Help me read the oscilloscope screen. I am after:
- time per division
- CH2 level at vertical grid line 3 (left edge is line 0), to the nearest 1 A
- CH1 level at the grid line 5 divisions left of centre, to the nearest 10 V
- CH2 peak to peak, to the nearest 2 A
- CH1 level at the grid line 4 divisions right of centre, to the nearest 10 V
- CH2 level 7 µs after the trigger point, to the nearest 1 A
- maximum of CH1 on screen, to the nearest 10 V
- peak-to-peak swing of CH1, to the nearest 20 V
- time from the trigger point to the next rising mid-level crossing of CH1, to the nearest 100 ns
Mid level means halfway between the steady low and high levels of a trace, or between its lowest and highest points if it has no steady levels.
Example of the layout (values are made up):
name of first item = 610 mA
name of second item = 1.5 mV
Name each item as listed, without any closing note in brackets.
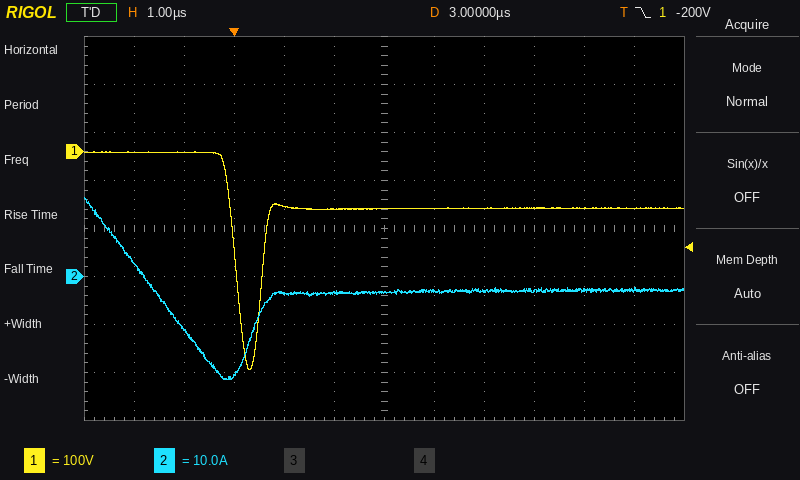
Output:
time per division = 1 µs
CH2 level at vertical grid line 3 (left edge is line 0), to the nearest 1 A = -21 A
CH1 level at the grid line 5 divisions left of centre, to the nearest 10 V = 0 V
CH2 peak to peak, to the nearest 2 A = 38 A
CH1 level at the grid line 4 divisions right of centre, to the nearest 10 V = -120 V
CH2 level 7 µs after the trigger point, to the nearest 1 A = -3 A
maximum of CH1 on screen, to the nearest 10 V = 0 V
peak-to-peak swing of CH1, to the nearest 20 V = 460 V
time from the trigger point to the next rising mid-level crossing of CH1, to the nearest 100 ns = 600 ns
